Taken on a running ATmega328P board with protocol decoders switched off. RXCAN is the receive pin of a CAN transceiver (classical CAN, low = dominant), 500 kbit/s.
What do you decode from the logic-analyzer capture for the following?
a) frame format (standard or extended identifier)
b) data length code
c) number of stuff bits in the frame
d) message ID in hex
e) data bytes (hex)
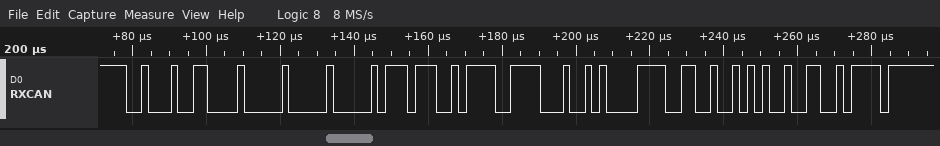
standard
8
3
0x226
00 07 72 F3 C4 A1 E6 4A
